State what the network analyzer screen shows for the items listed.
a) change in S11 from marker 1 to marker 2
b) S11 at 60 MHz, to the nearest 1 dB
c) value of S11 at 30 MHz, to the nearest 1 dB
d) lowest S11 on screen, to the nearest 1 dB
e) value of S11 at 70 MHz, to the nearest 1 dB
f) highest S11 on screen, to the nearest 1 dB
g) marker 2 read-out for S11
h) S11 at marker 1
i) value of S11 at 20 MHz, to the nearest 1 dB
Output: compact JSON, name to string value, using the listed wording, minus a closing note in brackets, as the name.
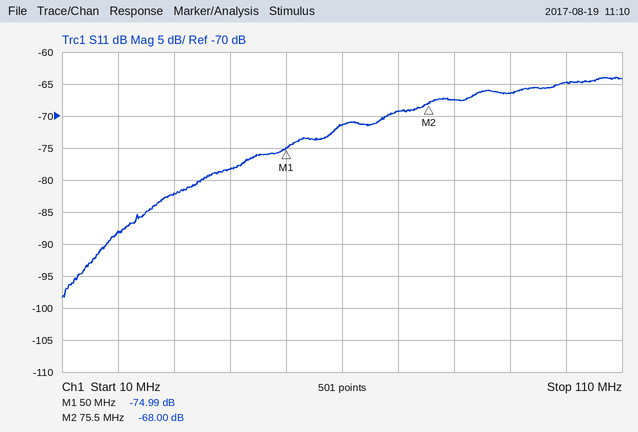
{"change in S11 from marker 1 to marker 2": "6.99 dB", "S11 at 60 MHz, to the nearest 1 dB": "-71 dB", "value of S11 at 30 MHz, to the nearest 1 dB": "-82 dB", "lowest S11 on screen, to the nearest 1 dB": "-98 dB", "value of S11 at 70 MHz, to the nearest 1 dB": "-69 dB", "highest S11 on screen, to the nearest 1 dB": "-64 dB", "marker 2 read-out for S11": "-68.00 dB", "S11 at marker 1": "-74.99 dB", "value of S11 at 20 MHz, to the nearest 1 dB": "-88 dB"}
